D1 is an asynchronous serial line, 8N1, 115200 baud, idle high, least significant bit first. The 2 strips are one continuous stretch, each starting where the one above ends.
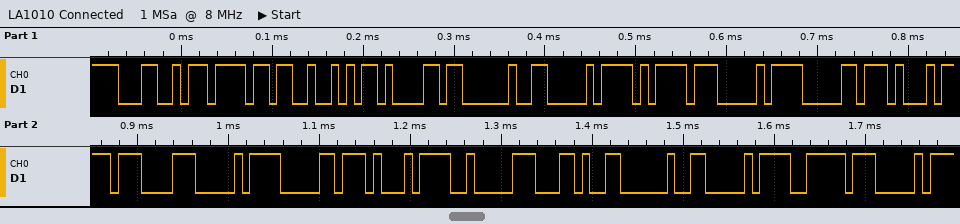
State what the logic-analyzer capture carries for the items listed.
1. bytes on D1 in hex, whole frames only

0x4C 0x6F 0x52 0x61 0x20 0xD0 0xBD 0xD0 0xB0 0xD1 0x87 0xD0 0xB0 0xD1 0x82 0x2C 0x20 0xD0 0xBE 0xD0
